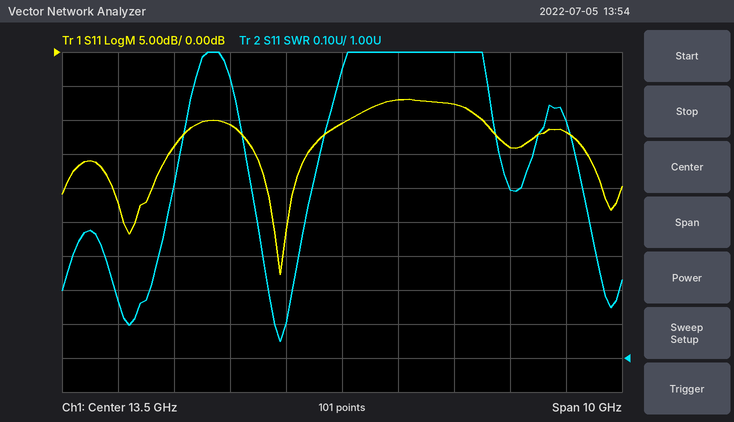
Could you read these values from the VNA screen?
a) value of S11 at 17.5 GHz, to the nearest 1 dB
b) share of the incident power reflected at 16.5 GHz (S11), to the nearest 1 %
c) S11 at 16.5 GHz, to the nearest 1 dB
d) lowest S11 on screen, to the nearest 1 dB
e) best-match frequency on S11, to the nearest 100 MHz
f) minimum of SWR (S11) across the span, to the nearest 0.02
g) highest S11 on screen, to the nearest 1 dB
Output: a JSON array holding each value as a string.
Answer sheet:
["-12 dB", "4 %", "-14 dB", "-33 dB", "12.4 GHz", "1.04", "-7 dB"]
